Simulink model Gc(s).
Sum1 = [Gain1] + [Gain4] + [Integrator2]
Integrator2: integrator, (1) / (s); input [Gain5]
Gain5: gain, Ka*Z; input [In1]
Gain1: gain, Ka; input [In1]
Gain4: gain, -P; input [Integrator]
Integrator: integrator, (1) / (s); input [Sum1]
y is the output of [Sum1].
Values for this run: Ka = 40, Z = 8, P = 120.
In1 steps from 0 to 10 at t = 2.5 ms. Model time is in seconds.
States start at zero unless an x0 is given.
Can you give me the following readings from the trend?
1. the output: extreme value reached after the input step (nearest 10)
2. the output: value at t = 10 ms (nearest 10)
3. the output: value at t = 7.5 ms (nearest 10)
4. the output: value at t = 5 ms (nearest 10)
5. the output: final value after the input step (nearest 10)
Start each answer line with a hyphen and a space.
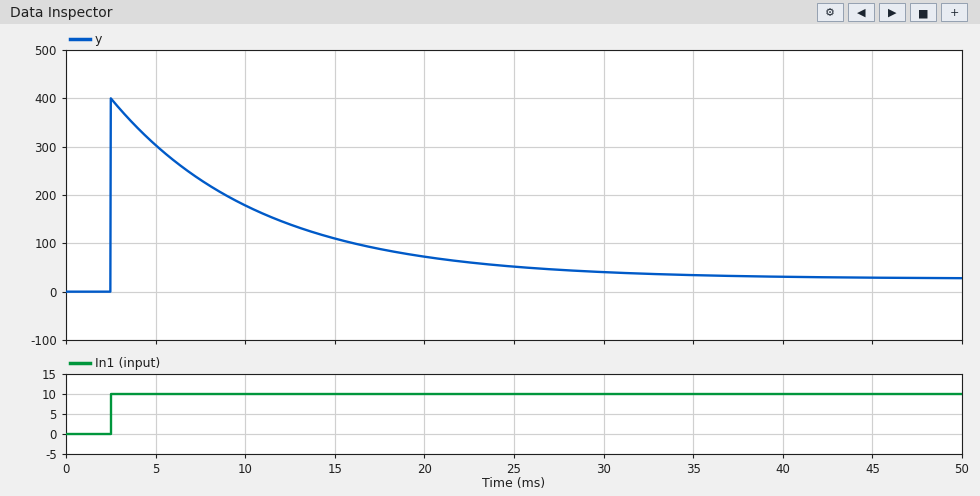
- 400
- 180
- 230
- 300
- 30
